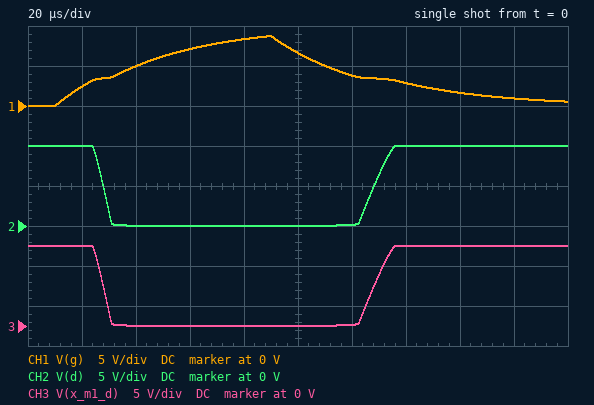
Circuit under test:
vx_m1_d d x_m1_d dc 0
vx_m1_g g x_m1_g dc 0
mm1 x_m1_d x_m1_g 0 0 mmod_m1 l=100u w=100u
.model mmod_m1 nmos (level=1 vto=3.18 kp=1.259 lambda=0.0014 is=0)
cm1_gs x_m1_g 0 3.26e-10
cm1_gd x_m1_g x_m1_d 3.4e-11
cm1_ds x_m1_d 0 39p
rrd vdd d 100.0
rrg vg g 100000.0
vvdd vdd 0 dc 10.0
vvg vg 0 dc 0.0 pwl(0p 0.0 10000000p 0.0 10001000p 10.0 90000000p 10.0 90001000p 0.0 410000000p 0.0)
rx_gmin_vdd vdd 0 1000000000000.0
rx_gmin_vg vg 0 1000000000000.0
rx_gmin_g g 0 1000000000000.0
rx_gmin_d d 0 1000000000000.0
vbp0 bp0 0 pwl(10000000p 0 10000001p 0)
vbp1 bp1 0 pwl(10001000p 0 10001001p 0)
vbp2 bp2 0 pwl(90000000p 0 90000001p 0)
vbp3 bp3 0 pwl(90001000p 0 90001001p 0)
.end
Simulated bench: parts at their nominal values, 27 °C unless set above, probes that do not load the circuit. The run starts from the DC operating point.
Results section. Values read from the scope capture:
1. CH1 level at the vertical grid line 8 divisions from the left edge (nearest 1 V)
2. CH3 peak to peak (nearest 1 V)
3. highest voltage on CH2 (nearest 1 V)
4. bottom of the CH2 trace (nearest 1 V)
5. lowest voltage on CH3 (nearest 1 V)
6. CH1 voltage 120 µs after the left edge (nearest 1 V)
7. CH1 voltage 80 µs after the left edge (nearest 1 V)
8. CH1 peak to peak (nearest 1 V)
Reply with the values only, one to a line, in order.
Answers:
2 V
10 V
10 V
0 V
0 V
4 V
8 V
9 V
